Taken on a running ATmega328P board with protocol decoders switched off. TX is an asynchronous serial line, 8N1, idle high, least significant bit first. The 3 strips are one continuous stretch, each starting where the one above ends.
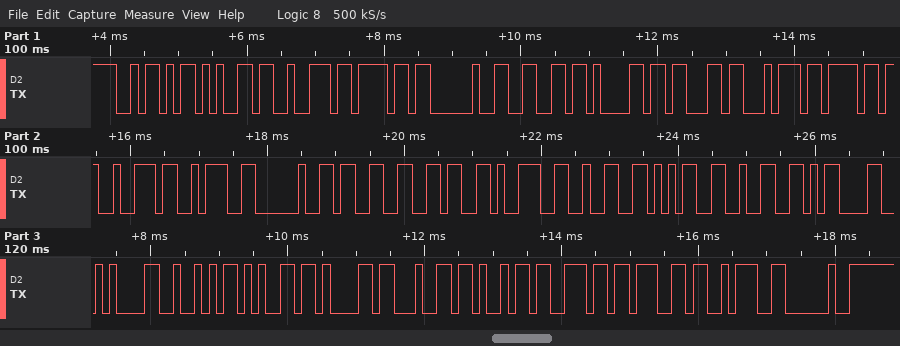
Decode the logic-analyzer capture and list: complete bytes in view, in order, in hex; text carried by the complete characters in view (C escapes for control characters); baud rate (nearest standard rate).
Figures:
5A 65 72 6F 20 66 61 63 74 6F 72 3A 20 33 36 39 32 35 32 0D 0A 52 65 61 64 69 6E 67 3A 20
"Zero factor: 369252\r\nReading: "
9600 baud
